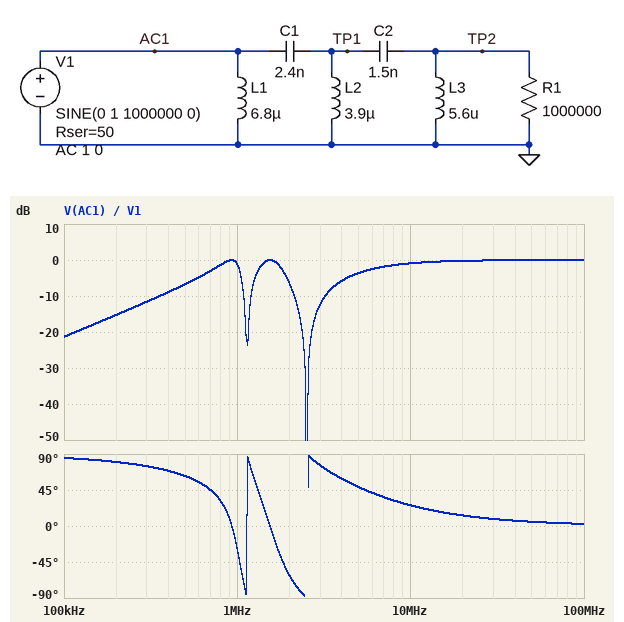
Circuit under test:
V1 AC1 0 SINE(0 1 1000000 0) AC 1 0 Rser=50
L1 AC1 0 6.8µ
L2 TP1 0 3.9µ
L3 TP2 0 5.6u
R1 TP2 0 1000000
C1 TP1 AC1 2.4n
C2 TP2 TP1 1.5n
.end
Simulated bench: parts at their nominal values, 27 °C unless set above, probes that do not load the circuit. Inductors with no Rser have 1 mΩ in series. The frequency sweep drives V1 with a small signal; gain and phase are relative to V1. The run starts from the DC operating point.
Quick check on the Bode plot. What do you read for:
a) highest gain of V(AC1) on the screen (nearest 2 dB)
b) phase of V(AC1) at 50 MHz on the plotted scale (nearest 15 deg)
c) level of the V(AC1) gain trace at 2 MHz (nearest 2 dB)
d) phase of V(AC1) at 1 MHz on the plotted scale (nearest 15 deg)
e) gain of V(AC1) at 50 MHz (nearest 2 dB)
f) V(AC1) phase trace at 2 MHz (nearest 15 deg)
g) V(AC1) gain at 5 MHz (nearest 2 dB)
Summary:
0 dB
0 deg
-6 dB
-30 deg
0 dB
-60 deg
-4 dB
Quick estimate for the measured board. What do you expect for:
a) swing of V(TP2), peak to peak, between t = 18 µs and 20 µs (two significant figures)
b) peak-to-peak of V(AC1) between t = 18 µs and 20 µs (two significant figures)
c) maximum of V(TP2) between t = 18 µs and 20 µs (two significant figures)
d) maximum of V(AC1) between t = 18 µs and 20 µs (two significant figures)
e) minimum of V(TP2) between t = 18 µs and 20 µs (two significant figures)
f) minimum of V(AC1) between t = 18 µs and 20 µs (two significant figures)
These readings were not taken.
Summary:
1.1 V
1.7 V
560 mV
870 mV
-560 mV
-870 mV
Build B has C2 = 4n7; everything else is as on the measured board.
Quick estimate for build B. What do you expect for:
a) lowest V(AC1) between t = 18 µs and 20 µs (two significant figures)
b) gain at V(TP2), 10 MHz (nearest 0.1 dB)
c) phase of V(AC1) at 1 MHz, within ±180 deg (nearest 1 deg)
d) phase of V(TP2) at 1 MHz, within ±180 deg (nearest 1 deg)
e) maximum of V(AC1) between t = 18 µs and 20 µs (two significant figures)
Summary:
-930 mV
-0.4 dB
22 deg
-158 deg
920 mV
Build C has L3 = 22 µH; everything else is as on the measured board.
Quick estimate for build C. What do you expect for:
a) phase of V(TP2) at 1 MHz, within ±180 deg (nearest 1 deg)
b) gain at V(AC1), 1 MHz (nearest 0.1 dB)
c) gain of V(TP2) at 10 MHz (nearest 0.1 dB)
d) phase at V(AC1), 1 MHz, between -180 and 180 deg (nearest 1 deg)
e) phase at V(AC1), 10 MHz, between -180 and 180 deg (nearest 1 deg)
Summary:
-168 deg
-0.2 dB
-0.2 dB
12 deg
20 deg
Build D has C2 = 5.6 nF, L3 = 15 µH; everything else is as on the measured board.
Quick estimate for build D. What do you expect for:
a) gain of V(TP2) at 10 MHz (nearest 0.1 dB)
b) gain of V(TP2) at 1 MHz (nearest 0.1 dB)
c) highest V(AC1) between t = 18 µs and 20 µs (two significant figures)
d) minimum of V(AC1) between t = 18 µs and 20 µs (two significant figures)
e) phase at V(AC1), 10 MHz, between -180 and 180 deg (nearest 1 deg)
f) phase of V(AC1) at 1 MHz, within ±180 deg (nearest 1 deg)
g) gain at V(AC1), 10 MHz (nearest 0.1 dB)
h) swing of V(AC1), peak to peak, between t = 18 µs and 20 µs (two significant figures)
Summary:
-0.3 dB
-5.6 dB
990 mV
-990 mV
21 deg
8 deg
-0.6 dB
2.0 V
